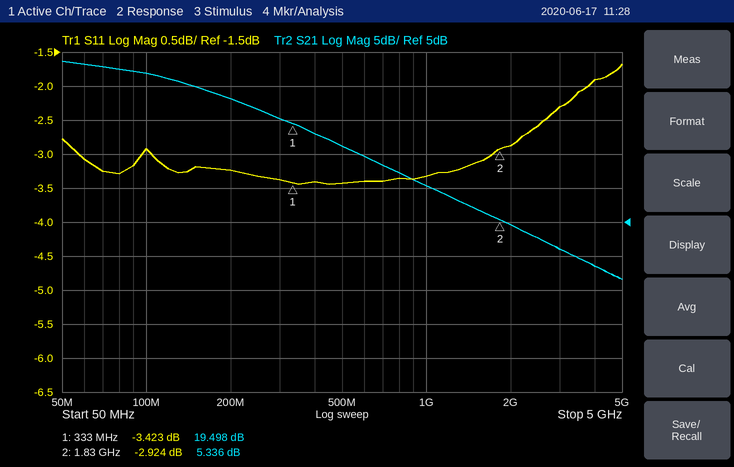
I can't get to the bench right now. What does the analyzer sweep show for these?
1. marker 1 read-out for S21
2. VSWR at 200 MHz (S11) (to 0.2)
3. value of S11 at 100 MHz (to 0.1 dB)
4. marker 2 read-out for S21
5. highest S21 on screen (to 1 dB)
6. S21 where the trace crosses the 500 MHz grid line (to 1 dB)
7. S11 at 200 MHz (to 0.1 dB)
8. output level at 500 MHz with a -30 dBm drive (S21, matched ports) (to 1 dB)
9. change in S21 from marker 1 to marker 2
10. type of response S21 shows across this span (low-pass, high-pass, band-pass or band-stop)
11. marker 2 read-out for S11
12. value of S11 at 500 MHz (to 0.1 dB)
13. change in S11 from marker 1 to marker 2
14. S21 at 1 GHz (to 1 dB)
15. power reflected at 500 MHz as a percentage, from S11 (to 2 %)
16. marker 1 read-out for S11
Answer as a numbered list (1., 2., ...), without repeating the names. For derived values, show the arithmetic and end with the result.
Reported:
1. 19.498 dB
2. |Γ| = 10^(-3.2/20) = 0.6918; VSWR = (1 + 0.6918)/(1 − 0.6918) ≈ 5.49, so 5.4 to the nearest 0.2
3. -2.9 dB
4. 5.336 dB
5. 29 dB
6. 16 dB
7. -3.2 dB
8. -30 dBm + (16 dB) = -14 dBm
9. 5.336 − (19.498) = -14.162 dB
10. low-pass
11. -2.924 dB
12. -3.4 dB
13. -2.924 − (-3.423) = 0.499 dB
14. 10 dB
15. 10^(-3.4/10) ≈ 46 %
16. -3.423 dB
